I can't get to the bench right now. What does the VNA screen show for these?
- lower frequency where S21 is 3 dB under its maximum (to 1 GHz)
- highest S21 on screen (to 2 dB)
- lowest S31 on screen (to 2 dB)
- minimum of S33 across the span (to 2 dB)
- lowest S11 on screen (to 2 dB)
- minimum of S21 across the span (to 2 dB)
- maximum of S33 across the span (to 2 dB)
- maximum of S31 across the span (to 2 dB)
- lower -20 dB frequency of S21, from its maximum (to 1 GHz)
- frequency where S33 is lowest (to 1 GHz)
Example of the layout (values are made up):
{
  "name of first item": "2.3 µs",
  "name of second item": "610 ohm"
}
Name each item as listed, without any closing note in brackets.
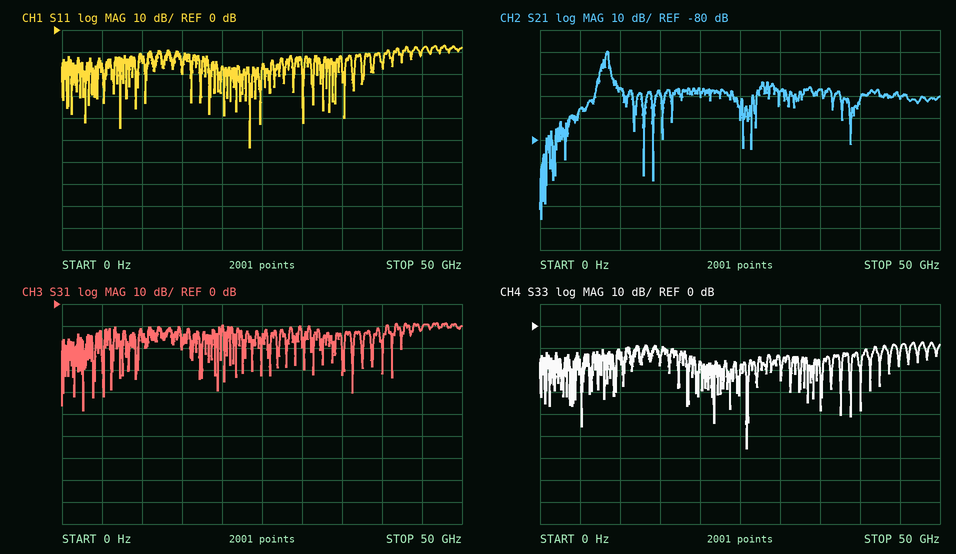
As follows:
{
  "lower frequency where S21 is 3 dB under its maximum": "8 GHz",
  "highest S21 on screen": "-40 dB",
  "lowest S31 on screen": "-48 dB",
  "minimum of S33 across the span": "-56 dB",
  "lowest S11 on screen": "-54 dB",
  "minimum of S21 across the span": "-116 dB",
  "maximum of S33 across the span": "-8 dB",
  "maximum of S31 across the span": "-8 dB",
  "lower -20 dB frequency of S21, from its maximum": "7 GHz",
  "frequency where S33 is lowest": "26 GHz"
}
